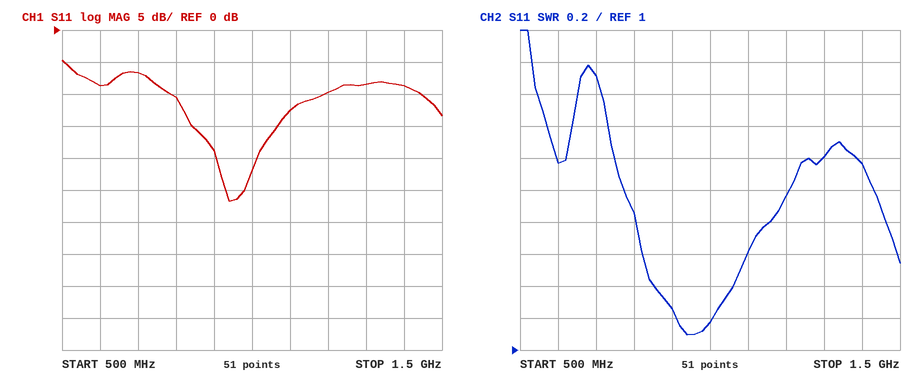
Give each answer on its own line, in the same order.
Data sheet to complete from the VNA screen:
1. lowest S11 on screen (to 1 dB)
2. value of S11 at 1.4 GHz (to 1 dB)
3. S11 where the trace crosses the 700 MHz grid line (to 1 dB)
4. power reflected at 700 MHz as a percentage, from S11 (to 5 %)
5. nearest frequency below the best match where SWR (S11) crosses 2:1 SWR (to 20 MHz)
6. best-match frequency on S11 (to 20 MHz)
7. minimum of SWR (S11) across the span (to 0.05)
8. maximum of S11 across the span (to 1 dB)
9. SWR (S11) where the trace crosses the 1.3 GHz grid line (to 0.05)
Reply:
-27 dB
-9 dB
-7 dB
20 %
780 MHz
940 MHz
1.10
-5 dB
2.20
